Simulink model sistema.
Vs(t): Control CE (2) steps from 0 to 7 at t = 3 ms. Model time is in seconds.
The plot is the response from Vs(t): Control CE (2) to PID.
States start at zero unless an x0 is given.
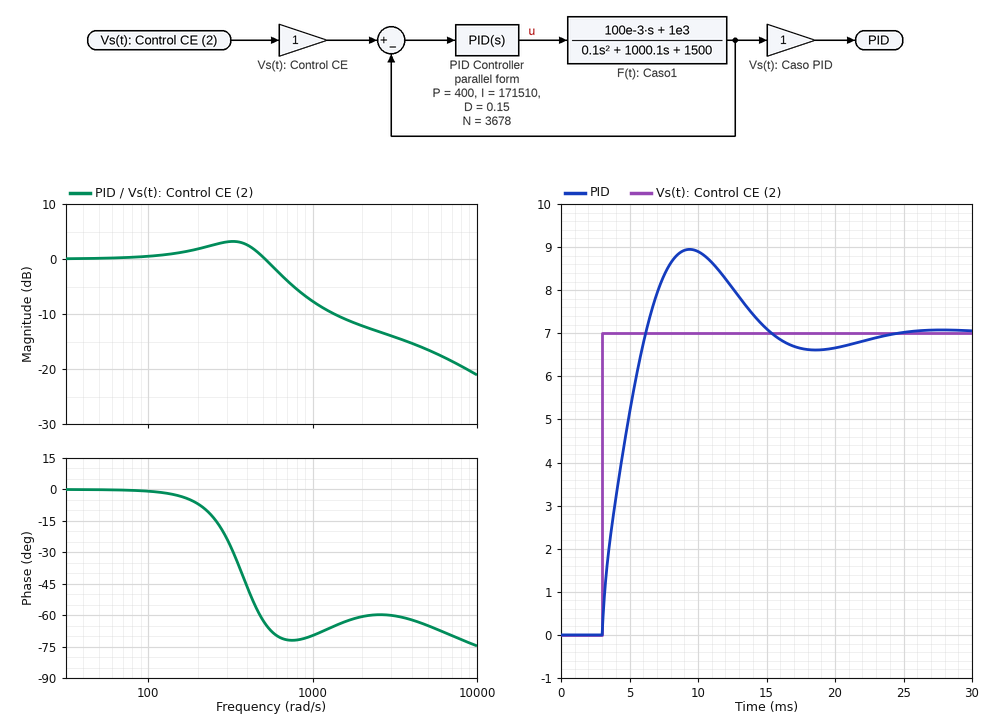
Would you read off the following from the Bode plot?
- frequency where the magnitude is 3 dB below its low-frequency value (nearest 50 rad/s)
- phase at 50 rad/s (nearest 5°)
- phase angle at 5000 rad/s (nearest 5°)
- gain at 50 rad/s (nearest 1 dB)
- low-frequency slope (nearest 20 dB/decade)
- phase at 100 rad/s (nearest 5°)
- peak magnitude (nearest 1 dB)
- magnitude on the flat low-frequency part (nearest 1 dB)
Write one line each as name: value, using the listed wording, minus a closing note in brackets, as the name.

frequency where the magnitude is 3 dB below its low-frequency value: 650 rad/s
phase at 50 rad/s: 0°
phase angle at 5000 rad/s: -65°
gain at 50 rad/s: 0 dB
low-frequency slope: 0 dB/decade
phase at 100 rad/s: 0°
peak magnitude: 3 dB
magnitude on the flat low-frequency part: 0 dB
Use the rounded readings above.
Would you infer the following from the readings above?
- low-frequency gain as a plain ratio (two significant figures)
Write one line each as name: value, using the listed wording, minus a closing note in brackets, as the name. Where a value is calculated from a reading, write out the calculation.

low-frequency gain as a plain ratio: 10^(0 / 20) = 1.0
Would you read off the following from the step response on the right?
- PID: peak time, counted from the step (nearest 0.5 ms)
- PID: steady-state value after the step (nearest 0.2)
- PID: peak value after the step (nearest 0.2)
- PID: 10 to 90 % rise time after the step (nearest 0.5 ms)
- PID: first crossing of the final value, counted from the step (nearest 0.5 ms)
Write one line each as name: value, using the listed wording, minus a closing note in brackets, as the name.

PID: peak time, counted from the step: 6.5 ms
PID: steady-state value after the step: 7.0
PID: peak value after the step: 9.0
PID: 10 to 90 % rise time after the step: 2.5 ms
PID: first crossing of the final value, counted from the step: 3.0 ms
